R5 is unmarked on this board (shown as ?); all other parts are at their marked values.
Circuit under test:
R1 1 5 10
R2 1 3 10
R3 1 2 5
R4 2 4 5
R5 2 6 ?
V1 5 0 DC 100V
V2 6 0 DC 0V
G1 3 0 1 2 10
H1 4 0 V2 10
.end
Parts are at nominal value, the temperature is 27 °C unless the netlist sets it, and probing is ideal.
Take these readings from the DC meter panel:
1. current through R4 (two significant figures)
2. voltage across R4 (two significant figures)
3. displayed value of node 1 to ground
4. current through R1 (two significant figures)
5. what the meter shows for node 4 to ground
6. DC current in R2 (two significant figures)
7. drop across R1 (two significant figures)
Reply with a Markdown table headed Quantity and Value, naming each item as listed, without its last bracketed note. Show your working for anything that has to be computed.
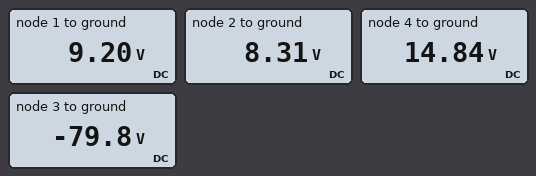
| Quantity | Value |
|---|---|
| current through R4 | (14.84 V - 8.31 V) / 5 Ω = 1.3 A |
| voltage across R4 | 14.84 V - 8.31 V = 6.5 V |
| displayed value of node 1 to ground | 9.20 V |
| current through R1 | (100 V - 9.2 V) / 10 Ω = 9.1 A |
| what the meter shows for node 4 to ground | 14.84 V |
| DC current in R2 | (9.2 V - (-79.8 V)) / 10 Ω = 8.9 A |
| drop across R1 | 100 V - 9.2 V = 91 V |
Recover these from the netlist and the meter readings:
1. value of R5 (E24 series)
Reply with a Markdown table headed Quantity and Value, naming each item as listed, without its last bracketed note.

| Quantity | Value |
|---|---|
| value of R5 | 5.6 Ω |
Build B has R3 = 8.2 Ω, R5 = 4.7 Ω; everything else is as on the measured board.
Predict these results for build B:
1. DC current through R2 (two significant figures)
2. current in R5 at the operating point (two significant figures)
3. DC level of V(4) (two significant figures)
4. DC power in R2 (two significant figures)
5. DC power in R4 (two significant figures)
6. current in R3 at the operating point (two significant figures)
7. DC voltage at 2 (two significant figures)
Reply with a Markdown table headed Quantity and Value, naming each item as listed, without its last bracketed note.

| Quantity | Value |
|---|---|
| DC current through R2 | 11 A |
| current in R5 at the operating point | 2.2 A |
| DC level of V(4) | -22 V |
| DC power in R2 | 1.2 kW |
| DC power in R4 | 27 W |
| current in R3 at the operating point | 130 mA |
| DC voltage at 2 | -10 V |
